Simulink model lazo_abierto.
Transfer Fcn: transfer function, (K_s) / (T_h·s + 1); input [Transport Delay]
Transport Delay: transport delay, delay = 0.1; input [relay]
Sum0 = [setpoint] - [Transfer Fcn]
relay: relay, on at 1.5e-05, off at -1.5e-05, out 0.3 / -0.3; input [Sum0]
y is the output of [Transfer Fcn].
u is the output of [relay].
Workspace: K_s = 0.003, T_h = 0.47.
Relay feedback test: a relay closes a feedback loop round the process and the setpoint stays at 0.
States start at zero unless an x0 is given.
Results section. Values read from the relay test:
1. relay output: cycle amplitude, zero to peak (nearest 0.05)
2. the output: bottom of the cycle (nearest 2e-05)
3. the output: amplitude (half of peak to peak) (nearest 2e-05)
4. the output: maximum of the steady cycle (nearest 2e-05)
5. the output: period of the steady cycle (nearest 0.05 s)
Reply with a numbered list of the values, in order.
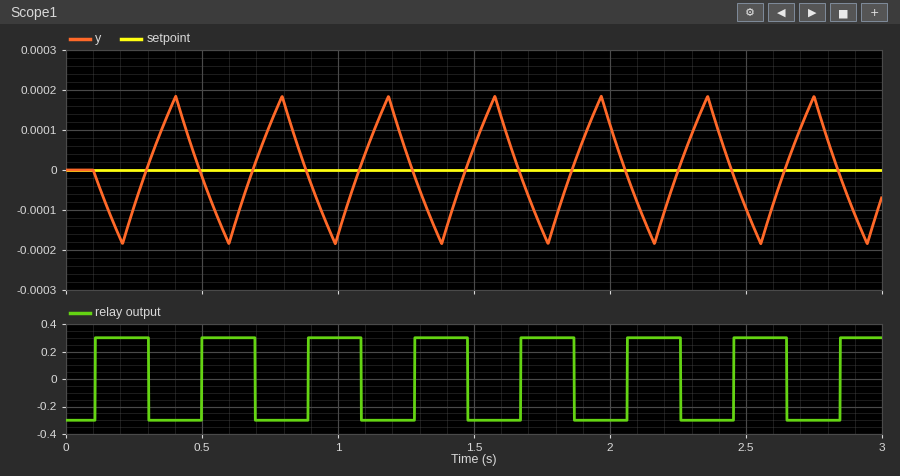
1. 0.30
2. -0.00018
3. 0.00018
4. 0.00018
5. 0.40 s
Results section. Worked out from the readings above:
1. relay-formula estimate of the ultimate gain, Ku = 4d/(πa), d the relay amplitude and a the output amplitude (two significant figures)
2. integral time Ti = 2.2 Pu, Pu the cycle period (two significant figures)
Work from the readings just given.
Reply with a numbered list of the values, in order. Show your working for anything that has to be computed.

1. 4 × 0.3 / (π × 0.00018) = 2100
2. 2.2 × 0.4 = 0.88 s
